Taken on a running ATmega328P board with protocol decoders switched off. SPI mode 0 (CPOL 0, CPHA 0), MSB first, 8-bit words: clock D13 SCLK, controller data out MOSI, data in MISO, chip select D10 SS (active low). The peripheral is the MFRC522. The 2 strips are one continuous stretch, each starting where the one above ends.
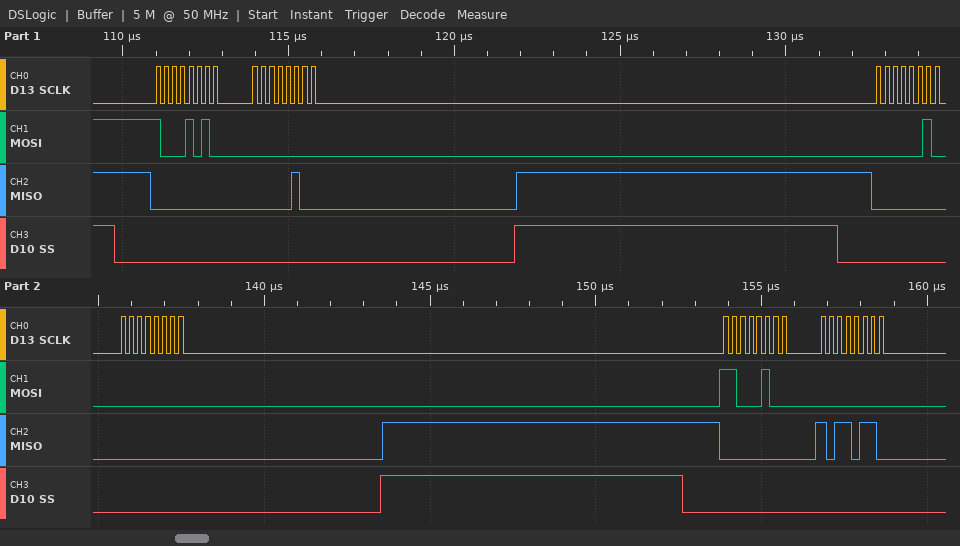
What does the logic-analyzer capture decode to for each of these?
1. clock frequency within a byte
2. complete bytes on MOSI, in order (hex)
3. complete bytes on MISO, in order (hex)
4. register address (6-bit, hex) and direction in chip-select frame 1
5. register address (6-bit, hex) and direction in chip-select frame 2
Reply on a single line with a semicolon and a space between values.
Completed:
4 MHz; 8A 00 02 00 C4 00; 00 04 00 00 00 B6; 0x05 read; 0x01 write
